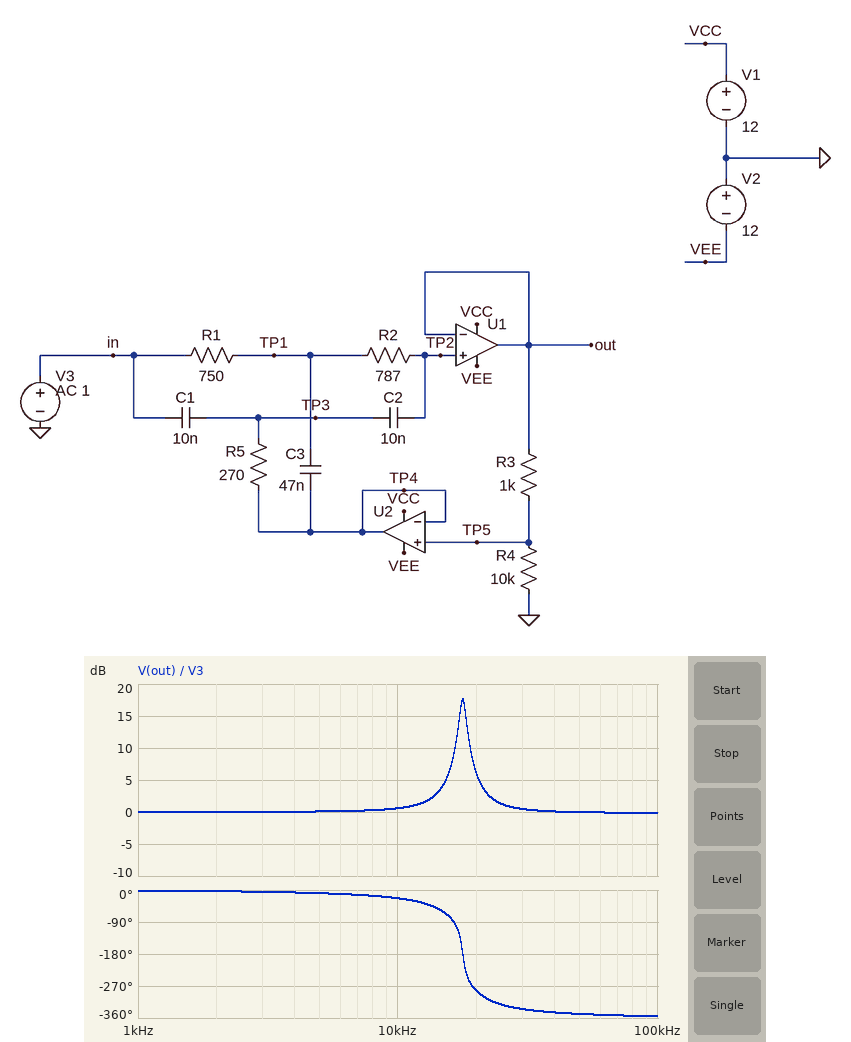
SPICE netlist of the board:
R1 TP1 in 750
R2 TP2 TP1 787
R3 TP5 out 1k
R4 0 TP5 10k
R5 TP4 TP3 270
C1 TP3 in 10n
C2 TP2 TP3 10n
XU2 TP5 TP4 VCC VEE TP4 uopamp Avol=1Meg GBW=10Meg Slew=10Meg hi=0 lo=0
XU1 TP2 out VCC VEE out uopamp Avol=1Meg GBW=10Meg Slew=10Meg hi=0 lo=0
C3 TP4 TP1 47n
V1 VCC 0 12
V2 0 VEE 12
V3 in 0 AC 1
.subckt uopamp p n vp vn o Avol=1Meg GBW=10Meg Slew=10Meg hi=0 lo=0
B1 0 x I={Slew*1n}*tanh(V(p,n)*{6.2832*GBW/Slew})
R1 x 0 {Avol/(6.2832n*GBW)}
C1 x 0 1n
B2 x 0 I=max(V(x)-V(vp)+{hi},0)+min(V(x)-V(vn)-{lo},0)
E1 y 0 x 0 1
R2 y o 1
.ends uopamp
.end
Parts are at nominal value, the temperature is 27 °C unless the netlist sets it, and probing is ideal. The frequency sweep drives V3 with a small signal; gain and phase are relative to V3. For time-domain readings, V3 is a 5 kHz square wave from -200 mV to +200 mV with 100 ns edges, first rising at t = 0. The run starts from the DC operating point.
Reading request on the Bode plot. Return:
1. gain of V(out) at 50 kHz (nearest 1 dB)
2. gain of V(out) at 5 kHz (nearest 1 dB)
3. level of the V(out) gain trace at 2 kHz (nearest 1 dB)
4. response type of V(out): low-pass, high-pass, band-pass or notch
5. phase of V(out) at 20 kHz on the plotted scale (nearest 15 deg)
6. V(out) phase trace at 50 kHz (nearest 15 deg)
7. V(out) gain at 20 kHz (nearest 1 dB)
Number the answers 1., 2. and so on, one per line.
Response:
1. 0 dB
2. 0 dB
3. 0 dB
4. band-pass
5. -285 deg
6. -345 deg
7. 6 dB
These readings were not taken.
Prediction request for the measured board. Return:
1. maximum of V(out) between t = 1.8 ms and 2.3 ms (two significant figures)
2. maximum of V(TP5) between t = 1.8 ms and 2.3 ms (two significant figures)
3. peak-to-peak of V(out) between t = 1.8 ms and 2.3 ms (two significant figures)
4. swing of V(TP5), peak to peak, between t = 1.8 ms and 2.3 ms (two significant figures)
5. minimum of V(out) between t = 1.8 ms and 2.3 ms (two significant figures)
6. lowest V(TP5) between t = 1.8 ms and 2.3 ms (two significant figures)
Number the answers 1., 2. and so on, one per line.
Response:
1. 340 mV
2. 310 mV
3. 670 mV
4. 610 mV
5. -340 mV
6. -310 mV
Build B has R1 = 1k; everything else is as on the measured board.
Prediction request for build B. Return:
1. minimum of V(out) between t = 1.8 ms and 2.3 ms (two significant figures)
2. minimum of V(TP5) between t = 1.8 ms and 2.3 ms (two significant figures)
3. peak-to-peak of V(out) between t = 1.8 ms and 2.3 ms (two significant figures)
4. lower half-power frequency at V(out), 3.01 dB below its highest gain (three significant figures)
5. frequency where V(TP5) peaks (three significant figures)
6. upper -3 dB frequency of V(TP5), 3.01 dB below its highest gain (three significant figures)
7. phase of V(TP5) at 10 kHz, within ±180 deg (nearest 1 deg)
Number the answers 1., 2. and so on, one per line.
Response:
1. -500 mV
2. -450 mV
3. 990 mV
4. 15.4 kHz
5. 16.1 kHz
6. 16.9 kHz
7. -32 deg
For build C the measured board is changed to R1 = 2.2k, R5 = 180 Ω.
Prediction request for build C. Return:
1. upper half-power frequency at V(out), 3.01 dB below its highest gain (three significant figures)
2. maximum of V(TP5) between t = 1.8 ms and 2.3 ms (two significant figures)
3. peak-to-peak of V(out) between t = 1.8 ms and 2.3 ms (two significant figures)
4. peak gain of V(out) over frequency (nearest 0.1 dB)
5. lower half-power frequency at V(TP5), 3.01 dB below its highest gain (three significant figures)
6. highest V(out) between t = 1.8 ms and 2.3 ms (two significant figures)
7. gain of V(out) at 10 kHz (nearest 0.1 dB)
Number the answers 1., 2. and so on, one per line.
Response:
1. 18.5 kHz
2. 380 mV
3. 830 mV
4. 6.0 dB
5. 11.9 kHz
6. 420 mV
7. 1.1 dB
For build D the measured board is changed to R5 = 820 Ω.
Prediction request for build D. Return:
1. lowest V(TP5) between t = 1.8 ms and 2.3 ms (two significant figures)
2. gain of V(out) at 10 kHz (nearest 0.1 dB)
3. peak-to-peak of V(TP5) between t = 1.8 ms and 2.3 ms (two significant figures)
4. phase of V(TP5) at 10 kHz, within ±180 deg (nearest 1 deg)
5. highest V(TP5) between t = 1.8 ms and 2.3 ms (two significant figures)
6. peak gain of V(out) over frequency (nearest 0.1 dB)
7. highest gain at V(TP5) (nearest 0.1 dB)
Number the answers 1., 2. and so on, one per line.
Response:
1. -250 mV
2. -1.0 dB
3. 500 mV
4. -33 deg
5. 250 mV
6. 0 dB
7. -0.8 dB
